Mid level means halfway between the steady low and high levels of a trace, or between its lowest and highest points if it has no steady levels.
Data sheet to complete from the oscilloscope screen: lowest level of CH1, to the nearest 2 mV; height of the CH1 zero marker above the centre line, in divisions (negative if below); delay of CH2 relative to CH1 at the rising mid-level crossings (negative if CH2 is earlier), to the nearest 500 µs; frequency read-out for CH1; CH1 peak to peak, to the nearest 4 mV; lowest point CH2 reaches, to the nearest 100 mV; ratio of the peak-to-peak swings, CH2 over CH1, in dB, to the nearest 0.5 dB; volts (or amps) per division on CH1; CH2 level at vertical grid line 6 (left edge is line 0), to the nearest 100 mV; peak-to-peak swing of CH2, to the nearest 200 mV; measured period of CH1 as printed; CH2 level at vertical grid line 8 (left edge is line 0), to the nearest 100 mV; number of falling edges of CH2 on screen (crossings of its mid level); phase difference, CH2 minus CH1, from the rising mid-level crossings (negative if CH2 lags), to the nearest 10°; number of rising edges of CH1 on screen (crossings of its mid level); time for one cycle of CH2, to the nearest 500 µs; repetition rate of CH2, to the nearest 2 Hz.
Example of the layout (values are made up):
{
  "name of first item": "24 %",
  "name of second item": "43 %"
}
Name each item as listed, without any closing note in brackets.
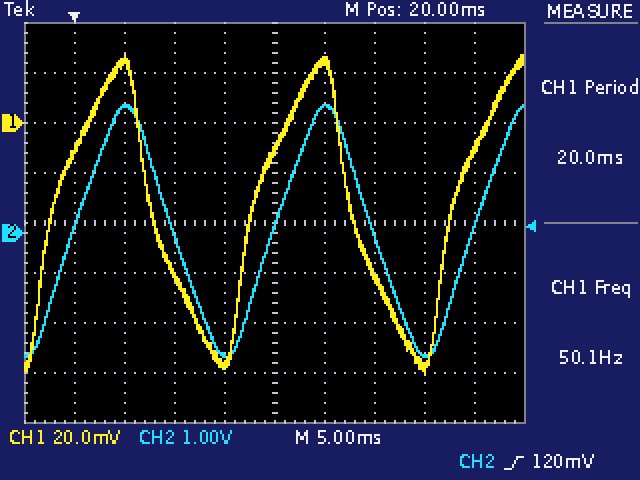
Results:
{
  "lowest level of CH1, to the nearest 2 mV": "-100 mV",
  "height of the CH1 zero marker above the centre line, in divisions": "+2.0 div",
  "delay of CH2 relative to CH1 at the rising mid-level crossings (negative if CH2 is earlier), to the nearest 500 µs": "+2.0 ms",
  "frequency read-out for CH1": "50.1 Hz",
  "CH1 peak to peak, to the nearest 4 mV": "128 mV",
  "lowest point CH2 reaches, to the nearest 100 mV": "-2.5 V",
  "ratio of the peak-to-peak swings, CH2 over CH1, in dB, to the nearest 0.5 dB": "32.0 dB",
  "volts (or amps) per division on CH1": "20 mV",
  "CH2 level at vertical grid line 6 (left edge is line 0), to the nearest 100 mV": "2.5 V",
  "peak-to-peak swing of CH2, to the nearest 200 mV": "5.0 V",
  "measured period of CH1 as printed": "20.0 ms",
  "CH2 level at vertical grid line 8 (left edge is line 0), to the nearest 100 mV": "-2.4 V",
  "number of falling edges of CH2 on screen": "2",
  "phase difference, CH2 minus CH1, from the rising mid-level crossings (negative if CH2 lags), to the nearest 10°": "-40°",
  "number of rising edges of CH1 on screen": "3",
  "time for one cycle of CH2, to the nearest 500 µs": "20.0 ms",
  "repetition rate of CH2, to the nearest 2 Hz": "50 Hz"
}
